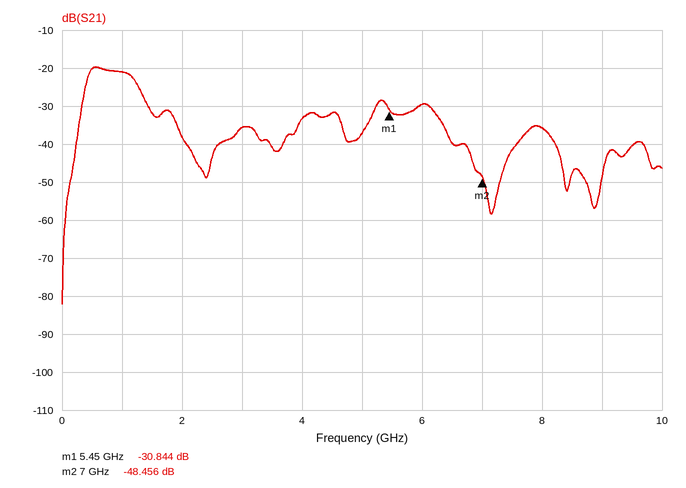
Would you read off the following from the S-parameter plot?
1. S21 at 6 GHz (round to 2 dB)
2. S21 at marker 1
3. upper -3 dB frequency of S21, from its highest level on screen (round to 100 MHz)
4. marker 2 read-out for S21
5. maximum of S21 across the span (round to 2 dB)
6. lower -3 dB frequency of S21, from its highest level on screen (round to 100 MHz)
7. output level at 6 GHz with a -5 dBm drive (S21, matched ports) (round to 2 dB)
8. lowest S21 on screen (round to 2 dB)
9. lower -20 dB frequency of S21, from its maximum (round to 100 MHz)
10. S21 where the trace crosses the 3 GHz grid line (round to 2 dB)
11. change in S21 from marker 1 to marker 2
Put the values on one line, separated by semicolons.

-30 dB; -30.844 dB; 1.2 GHz; -48.456 dB; -20 dB; 400 MHz; -34 dBm; -82 dB; 200 MHz; -36 dB; -17.612 dB
